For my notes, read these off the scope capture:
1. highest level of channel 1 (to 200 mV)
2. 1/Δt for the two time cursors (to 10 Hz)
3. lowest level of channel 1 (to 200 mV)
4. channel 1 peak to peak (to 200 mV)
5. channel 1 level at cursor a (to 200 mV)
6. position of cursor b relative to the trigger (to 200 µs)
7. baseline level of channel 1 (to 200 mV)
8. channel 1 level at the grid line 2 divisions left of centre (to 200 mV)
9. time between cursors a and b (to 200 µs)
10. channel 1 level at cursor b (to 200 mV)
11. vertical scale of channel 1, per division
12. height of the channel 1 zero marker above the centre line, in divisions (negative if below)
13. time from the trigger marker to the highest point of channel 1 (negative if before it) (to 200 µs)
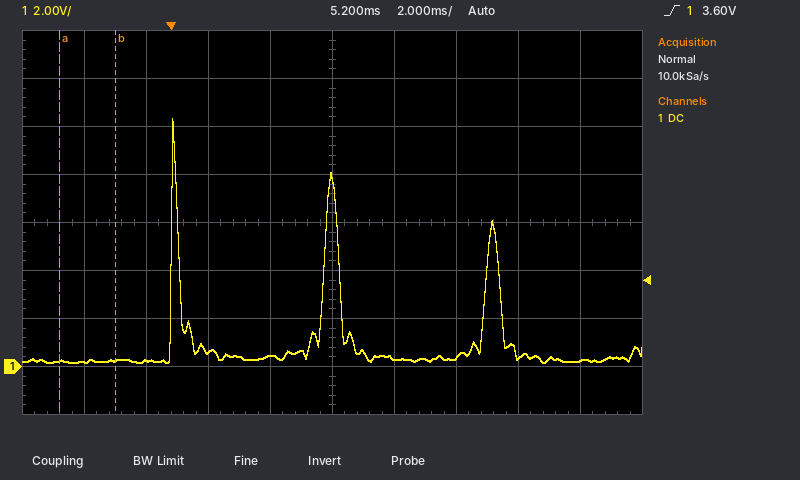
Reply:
10.4 V
560 Hz
200 mV
10.2 V
200 mV
-1.8 ms
200 mV
600 mV
1.8 ms
200 mV
2 V
-3.0 div
0.0 ms
